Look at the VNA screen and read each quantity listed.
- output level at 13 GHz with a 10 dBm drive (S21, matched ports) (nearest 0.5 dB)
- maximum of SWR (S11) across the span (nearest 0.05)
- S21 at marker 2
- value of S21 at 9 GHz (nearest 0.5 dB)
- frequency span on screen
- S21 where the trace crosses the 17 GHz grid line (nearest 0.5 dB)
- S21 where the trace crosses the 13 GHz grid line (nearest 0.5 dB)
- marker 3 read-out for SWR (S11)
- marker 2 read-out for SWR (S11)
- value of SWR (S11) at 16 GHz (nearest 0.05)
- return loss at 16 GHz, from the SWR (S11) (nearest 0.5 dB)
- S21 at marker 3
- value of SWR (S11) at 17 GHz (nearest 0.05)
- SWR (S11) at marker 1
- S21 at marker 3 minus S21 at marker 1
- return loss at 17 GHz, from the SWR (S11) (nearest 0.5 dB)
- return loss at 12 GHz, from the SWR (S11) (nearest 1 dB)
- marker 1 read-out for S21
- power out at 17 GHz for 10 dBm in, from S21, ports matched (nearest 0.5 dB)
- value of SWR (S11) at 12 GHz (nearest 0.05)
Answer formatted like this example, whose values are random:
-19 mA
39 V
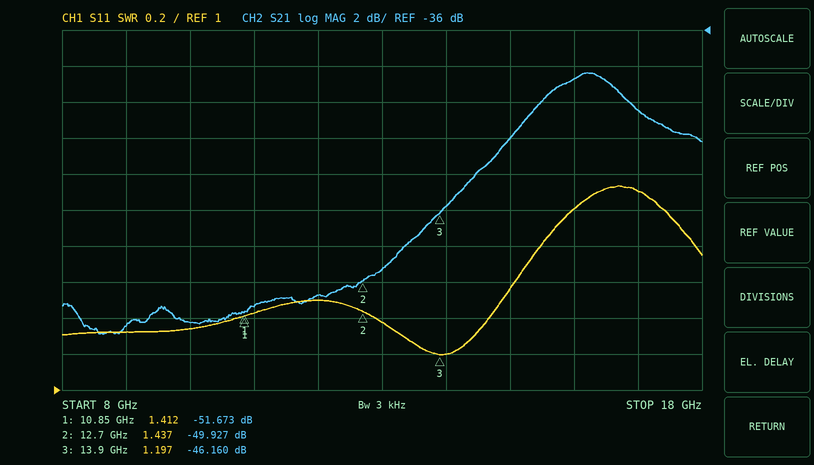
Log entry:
-39.5 dBm
2.15
-49.927 dB
-52.5 dB
10 GHz
-40.5 dB
-49.5 dB
1.197
1.437
2.00
9.5 dB
-46.160 dB
2.10
1.412
5.513 dB
9.0 dB
14 dB
-51.673 dB
-30.5 dBm
1.50
